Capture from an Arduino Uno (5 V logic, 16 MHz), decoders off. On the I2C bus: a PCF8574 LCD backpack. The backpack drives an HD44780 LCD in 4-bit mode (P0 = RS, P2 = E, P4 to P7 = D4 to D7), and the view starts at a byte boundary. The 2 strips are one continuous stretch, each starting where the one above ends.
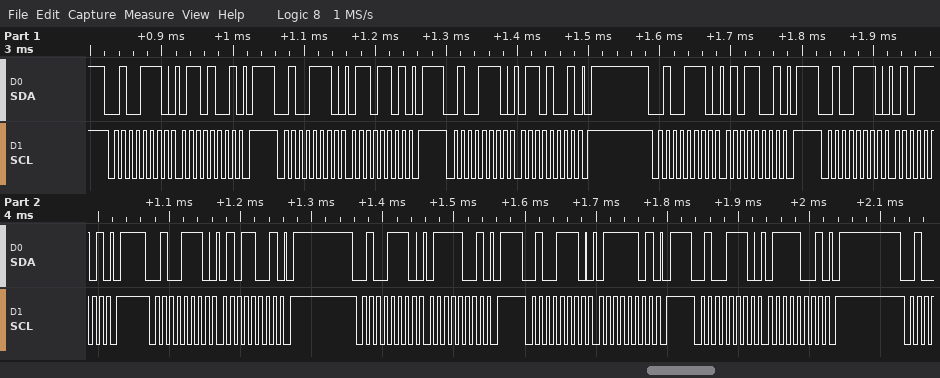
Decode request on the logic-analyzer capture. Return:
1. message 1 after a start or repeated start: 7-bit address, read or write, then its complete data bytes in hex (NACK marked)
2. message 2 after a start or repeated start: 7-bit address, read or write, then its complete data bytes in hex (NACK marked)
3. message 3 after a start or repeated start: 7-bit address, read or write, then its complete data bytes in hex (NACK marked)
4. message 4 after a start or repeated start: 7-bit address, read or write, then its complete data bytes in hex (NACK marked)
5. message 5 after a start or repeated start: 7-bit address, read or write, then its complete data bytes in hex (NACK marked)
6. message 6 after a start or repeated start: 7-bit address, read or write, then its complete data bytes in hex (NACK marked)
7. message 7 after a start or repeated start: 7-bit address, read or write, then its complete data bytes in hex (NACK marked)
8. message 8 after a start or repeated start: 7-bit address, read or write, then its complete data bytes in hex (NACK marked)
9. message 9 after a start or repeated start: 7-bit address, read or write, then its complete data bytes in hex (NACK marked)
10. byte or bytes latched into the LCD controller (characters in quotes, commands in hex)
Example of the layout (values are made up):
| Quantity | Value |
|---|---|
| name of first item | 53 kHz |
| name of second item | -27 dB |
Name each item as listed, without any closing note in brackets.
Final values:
| Quantity | Value |
|---|---|
| message 1 after a start or repeated start: 7-bit address, read or write, then its complete data bytes in hex | 0x27 write: 69 |
| message 2 after a start or repeated start: 7-bit address, read or write, then its complete data bytes in hex | 0x27 write: 6D |
| message 3 after a start or repeated start: 7-bit address, read or write, then its complete data bytes in hex | 0x27 write: 69 |
| message 4 after a start or repeated start: 7-bit address, read or write, then its complete data bytes in hex | 0x27 write: 59 |
| message 5 after a start or repeated start: 7-bit address, read or write, then its complete data bytes in hex | 0x27 write: 5D |
| message 6 after a start or repeated start: 7-bit address, read or write, then its complete data bytes in hex | 0x27 write: 59 |
| message 7 after a start or repeated start: 7-bit address, read or write, then its complete data bytes in hex | 0x27 write: 79 |
| message 8 after a start or repeated start: 7-bit address, read or write, then its complete data bytes in hex | 0x27 write: 7D |
| message 9 after a start or repeated start: 7-bit address, read or write, then its complete data bytes in hex | 0x27 write: 79 |
| byte or bytes latched into the LCD controller | 'e' |
